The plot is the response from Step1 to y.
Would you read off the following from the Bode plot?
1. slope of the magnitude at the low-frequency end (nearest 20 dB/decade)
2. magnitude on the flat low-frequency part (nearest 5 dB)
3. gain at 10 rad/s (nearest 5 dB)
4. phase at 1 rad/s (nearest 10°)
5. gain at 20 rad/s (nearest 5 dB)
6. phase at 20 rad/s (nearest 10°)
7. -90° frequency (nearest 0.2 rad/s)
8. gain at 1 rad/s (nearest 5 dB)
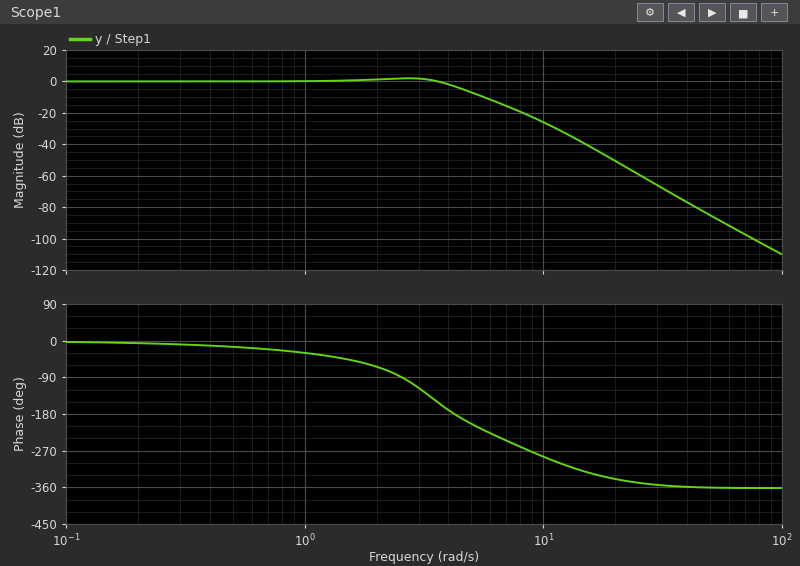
0 dB/decade
0 dB
-25 dB
-30°
-50 dB
-340°
2.6 rad/s
0 dB
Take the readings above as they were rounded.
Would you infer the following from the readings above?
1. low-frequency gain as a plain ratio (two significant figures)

1.0
